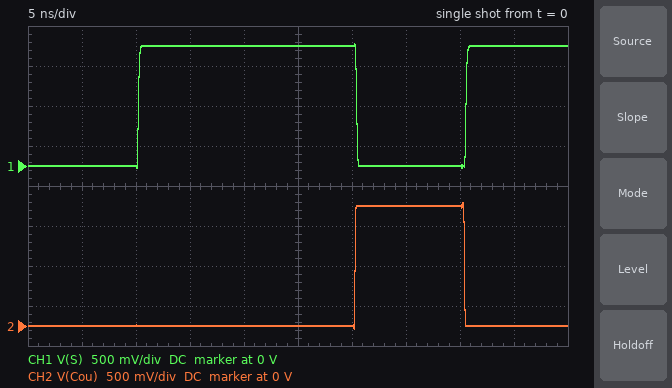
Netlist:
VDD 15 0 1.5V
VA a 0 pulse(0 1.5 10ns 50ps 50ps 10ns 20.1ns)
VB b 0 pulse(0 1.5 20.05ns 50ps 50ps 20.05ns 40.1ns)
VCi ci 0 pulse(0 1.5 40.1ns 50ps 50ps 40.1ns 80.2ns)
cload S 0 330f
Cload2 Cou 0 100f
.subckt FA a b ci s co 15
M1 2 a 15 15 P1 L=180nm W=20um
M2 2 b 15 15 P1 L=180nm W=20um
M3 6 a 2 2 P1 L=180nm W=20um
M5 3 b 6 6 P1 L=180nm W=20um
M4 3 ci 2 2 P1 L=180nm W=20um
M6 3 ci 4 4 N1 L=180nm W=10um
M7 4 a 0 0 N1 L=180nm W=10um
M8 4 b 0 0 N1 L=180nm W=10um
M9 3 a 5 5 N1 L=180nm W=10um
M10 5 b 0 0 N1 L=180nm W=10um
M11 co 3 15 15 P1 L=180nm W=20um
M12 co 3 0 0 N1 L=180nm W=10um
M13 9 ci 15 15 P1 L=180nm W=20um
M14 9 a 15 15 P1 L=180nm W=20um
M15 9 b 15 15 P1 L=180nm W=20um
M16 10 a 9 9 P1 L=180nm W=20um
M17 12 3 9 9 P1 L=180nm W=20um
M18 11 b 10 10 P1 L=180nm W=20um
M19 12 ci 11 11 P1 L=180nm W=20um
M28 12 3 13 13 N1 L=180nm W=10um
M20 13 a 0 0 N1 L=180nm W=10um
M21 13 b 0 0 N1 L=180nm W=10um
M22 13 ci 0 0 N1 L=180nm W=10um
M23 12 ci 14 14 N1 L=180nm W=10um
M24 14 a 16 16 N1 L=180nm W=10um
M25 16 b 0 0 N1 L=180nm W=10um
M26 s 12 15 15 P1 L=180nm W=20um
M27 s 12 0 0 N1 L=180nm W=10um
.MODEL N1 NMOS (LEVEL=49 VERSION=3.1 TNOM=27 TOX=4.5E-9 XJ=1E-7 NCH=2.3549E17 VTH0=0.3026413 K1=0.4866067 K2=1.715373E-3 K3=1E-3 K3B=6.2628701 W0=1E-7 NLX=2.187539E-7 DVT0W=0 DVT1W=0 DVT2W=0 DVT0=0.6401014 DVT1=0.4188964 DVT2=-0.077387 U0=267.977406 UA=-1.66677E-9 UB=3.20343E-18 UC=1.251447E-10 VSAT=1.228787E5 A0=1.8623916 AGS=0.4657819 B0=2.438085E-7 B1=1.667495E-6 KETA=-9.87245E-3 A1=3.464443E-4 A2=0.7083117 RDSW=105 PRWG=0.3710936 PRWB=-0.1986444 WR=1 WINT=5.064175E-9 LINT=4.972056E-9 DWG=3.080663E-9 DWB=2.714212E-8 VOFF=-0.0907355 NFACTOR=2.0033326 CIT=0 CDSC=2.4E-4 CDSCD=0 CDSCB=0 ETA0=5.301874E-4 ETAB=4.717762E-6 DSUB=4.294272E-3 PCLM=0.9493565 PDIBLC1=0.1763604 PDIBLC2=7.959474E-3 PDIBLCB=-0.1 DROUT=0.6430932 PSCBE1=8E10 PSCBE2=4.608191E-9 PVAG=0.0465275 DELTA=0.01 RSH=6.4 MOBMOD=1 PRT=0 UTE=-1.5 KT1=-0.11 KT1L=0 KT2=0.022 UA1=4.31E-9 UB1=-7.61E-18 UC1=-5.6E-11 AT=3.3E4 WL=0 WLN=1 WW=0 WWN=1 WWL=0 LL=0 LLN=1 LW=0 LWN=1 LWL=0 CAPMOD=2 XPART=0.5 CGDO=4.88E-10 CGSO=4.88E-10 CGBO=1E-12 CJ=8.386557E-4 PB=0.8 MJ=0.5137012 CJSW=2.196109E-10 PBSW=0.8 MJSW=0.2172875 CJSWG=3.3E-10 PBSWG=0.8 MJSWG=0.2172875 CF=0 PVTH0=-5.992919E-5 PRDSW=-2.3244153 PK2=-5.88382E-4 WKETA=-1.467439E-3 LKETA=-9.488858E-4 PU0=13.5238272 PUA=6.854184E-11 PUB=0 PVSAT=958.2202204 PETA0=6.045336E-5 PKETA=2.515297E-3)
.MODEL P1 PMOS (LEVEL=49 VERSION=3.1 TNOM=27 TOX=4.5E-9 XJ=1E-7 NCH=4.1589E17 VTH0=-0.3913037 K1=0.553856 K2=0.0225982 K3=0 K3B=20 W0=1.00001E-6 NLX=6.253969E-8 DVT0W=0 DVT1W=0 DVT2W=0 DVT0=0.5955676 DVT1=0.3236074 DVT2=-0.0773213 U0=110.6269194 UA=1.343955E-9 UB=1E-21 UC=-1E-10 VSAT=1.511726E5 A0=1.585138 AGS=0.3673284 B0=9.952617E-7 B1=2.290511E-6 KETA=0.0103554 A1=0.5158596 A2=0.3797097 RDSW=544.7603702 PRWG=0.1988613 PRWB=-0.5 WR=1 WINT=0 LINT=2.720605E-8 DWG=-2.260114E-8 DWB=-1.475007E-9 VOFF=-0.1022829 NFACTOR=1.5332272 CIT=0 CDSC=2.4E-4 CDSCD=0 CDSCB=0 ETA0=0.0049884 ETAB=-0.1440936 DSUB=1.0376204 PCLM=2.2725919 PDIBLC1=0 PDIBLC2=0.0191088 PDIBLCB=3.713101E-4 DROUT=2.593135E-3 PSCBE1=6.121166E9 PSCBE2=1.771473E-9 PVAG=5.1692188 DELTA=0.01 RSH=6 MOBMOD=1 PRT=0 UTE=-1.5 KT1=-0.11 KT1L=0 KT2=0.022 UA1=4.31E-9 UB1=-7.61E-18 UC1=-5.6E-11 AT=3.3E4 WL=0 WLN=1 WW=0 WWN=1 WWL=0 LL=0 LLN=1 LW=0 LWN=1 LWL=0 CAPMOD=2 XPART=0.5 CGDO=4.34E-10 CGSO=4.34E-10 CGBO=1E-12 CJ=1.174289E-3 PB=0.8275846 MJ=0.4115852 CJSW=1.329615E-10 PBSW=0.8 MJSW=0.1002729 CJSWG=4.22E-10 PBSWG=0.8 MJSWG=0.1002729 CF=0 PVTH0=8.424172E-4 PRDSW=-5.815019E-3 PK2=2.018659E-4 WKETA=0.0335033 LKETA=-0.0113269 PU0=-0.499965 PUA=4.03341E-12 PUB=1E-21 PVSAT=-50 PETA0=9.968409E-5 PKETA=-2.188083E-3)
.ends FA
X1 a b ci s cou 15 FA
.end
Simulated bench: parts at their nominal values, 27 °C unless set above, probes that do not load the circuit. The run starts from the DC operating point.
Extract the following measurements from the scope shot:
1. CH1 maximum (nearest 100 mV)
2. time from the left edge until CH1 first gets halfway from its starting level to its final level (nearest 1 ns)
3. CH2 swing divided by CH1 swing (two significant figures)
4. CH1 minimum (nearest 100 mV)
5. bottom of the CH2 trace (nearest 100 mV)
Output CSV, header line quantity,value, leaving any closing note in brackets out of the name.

quantity,value
CH1 maximum,1.5 V
time from the left edge until CH1 first gets halfway from its starting level to its final level,10 ns
CH2 swing divided by CH1 swing,1.0
CH1 minimum,0 V
bottom of the CH2 trace,0 V
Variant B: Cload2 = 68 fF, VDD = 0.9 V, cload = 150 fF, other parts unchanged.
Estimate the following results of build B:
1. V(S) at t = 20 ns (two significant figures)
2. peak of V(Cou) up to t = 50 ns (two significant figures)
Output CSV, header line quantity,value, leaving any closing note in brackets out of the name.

quantity,value
V(S) at t = 20 ns,900 mV
peak of V(Cou) up to t = 50 ns,940 mV
